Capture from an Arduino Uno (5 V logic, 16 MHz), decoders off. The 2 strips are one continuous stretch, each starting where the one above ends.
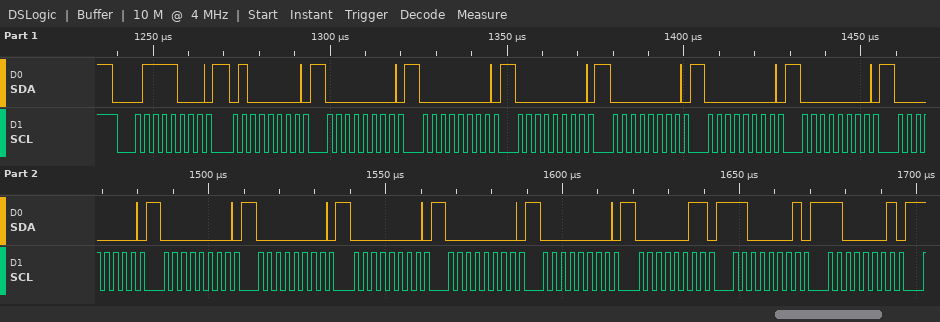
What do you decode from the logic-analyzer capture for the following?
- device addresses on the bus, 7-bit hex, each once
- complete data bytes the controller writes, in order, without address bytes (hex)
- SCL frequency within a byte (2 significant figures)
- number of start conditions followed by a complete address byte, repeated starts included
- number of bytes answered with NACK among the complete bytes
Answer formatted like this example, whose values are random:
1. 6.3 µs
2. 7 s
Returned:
1. 0x3C
2. 40 00 00 00 00 00 00 00 00 00 00 00 00 03 C1 C1
3. 400 kHz
4. 1
5. 0
